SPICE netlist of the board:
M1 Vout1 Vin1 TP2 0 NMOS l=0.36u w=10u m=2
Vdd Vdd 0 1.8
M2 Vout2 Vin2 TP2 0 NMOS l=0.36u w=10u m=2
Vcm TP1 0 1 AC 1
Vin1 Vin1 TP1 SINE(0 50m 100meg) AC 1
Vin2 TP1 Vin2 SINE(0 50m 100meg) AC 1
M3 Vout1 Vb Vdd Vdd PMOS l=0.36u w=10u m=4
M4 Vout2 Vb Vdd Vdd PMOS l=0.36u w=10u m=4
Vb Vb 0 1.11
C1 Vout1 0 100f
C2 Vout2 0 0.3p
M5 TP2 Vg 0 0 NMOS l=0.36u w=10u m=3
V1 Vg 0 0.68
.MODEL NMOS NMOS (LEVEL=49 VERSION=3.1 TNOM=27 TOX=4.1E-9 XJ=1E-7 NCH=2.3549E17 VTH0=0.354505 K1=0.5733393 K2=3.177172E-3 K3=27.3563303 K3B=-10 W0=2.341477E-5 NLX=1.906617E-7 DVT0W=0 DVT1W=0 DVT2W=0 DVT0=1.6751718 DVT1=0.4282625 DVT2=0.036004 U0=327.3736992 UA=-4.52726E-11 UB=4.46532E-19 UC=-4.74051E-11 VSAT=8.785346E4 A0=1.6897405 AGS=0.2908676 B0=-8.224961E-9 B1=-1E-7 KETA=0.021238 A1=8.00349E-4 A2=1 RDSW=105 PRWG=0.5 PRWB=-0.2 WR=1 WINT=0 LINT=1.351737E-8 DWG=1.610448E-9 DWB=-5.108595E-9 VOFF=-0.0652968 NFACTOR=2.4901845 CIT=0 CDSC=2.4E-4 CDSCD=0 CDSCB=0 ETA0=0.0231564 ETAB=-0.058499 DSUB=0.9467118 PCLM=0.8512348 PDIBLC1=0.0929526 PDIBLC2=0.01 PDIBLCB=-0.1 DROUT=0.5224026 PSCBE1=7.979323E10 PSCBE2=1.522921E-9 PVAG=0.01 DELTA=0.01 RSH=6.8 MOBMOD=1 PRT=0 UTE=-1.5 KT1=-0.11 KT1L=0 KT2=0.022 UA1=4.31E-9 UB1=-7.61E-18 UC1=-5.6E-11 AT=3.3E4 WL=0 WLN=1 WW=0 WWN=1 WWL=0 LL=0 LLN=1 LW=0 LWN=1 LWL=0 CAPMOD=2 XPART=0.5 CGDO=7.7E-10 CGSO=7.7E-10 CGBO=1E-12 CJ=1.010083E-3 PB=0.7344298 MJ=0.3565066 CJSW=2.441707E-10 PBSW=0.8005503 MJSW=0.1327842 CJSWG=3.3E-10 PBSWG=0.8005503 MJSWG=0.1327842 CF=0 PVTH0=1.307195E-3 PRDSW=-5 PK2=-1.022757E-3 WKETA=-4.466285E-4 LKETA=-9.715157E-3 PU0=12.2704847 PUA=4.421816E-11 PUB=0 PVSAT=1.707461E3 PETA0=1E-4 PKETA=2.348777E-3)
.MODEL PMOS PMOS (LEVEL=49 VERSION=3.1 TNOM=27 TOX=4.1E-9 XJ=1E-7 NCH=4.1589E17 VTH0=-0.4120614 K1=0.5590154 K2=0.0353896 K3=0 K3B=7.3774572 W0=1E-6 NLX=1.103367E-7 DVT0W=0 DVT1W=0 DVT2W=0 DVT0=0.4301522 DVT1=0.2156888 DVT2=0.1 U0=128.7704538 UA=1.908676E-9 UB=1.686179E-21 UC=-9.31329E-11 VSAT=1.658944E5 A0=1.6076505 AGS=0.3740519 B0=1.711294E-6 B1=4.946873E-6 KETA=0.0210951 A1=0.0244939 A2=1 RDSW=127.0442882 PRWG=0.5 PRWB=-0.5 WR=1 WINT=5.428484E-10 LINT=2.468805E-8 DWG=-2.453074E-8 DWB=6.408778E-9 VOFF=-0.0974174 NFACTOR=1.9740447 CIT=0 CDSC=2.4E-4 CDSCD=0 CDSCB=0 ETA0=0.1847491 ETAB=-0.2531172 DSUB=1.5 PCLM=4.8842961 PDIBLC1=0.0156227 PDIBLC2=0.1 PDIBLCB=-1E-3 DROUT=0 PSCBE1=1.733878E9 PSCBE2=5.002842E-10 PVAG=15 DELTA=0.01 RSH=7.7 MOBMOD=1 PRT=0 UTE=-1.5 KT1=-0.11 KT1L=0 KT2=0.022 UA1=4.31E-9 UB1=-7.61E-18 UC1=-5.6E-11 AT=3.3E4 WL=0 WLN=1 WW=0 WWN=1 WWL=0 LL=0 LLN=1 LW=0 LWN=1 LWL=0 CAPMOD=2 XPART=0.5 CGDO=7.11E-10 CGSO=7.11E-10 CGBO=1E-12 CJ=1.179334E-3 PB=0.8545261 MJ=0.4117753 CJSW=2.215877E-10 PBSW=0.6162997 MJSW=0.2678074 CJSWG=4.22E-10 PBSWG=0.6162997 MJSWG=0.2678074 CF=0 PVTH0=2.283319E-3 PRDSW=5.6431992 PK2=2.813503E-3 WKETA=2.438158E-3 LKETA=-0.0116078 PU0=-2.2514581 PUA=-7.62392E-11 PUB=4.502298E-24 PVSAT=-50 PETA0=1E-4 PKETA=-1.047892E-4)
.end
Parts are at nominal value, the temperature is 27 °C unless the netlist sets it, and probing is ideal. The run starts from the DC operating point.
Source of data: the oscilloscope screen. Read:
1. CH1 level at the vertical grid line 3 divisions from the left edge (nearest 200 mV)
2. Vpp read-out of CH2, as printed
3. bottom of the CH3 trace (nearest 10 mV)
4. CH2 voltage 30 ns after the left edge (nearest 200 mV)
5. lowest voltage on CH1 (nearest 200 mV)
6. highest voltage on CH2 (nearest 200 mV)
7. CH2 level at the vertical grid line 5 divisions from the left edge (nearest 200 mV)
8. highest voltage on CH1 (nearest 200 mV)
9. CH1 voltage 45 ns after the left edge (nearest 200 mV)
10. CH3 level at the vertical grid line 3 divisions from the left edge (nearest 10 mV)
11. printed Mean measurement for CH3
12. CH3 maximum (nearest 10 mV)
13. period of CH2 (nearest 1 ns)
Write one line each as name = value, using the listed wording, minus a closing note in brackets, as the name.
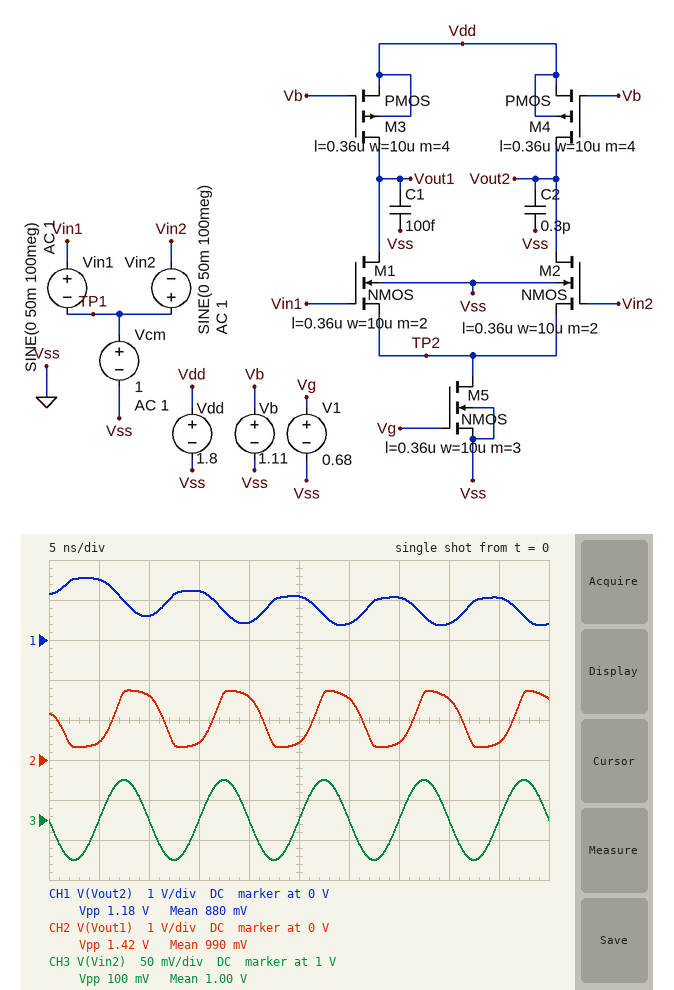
CH1 level at the vertical grid line 3 divisions from the left edge = 1.2 V
Vpp read-out of CH2, as printed = 1.42 V
bottom of the CH3 trace = 950 mV
CH2 voltage 30 ns after the left edge = 1.6 V
lowest voltage on CH1 = 400 mV
highest voltage on CH2 = 1.8 V
CH2 level at the vertical grid line 5 divisions from the left edge = 400 mV
highest voltage on CH1 = 1.6 V
CH1 voltage 45 ns after the left edge = 1.0 V
CH3 level at the vertical grid line 3 divisions from the left edge = 1.00 V
printed Mean measurement for CH3 = 1.00 V
CH3 maximum = 1.05 V
period of CH2 = 10 ns
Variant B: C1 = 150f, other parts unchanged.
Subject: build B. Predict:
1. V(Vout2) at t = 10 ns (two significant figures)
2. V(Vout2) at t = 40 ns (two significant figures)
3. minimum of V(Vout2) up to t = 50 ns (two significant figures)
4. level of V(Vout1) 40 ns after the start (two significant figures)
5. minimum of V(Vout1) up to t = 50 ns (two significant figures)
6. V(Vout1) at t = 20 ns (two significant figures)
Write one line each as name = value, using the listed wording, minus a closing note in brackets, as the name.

V(Vout2) at t = 10 ns = 620 mV
V(Vout2) at t = 40 ns = 440 mV
minimum of V(Vout2) up to t = 50 ns = 410 mV
level of V(Vout1) 40 ns after the start = 1.6 V
minimum of V(Vout1) up to t = 50 ns = 330 mV
V(Vout1) at t = 20 ns = 1.6 V
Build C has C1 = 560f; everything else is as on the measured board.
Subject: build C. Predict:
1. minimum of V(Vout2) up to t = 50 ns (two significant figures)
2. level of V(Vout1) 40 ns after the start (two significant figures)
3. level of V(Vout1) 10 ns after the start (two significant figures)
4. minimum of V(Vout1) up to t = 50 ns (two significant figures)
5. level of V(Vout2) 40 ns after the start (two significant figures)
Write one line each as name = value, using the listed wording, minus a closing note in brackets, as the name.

minimum of V(Vout2) up to t = 50 ns = 610 mV
level of V(Vout1) 40 ns after the start = 1.4 V
level of V(Vout1) 10 ns after the start = 1.3 V
minimum of V(Vout1) up to t = 50 ns = 650 mV
level of V(Vout2) 40 ns after the start = 620 mV
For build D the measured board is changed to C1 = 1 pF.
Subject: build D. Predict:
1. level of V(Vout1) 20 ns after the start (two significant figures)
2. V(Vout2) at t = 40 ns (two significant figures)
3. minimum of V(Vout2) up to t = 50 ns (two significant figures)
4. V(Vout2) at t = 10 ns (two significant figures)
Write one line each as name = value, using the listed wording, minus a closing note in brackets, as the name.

level of V(Vout1) 20 ns after the start = 1.2 V
V(Vout2) at t = 40 ns = 620 mV
minimum of V(Vout2) up to t = 50 ns = 610 mV
V(Vout2) at t = 10 ns = 650 mV
